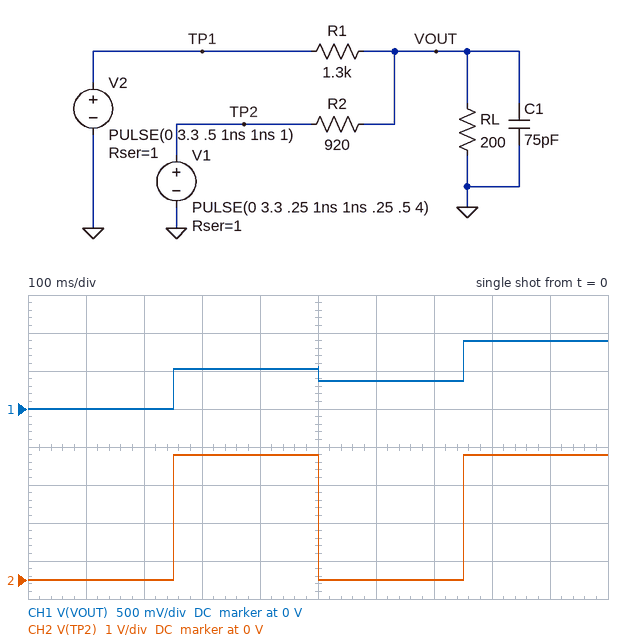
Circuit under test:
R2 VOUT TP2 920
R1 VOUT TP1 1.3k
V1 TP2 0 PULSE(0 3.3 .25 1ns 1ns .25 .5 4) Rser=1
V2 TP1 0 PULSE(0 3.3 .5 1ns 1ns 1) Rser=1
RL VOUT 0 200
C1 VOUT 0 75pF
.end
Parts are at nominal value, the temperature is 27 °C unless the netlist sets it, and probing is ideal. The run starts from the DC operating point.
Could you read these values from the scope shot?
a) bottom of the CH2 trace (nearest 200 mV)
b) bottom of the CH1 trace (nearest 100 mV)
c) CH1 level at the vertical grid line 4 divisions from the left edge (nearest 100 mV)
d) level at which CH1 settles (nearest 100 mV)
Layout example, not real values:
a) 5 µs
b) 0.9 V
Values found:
a) 0 V
b) 0 V
c) 500 mV
d) 900 mV
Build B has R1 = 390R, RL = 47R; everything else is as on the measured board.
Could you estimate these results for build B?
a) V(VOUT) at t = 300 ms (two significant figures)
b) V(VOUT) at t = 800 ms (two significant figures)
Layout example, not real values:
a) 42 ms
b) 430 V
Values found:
a) 140 mV
b) 480 mV
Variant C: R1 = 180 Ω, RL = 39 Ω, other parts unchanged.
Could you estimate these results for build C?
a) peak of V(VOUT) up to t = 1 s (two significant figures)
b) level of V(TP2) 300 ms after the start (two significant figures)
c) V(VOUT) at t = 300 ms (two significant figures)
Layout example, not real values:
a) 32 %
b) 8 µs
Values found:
a) 680 mV
b) 3.3 V
c) 110 mV
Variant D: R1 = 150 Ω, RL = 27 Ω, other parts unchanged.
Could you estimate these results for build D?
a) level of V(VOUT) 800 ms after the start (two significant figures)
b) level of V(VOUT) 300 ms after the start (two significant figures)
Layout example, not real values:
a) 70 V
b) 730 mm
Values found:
a) 570 mV
b) 80 mV
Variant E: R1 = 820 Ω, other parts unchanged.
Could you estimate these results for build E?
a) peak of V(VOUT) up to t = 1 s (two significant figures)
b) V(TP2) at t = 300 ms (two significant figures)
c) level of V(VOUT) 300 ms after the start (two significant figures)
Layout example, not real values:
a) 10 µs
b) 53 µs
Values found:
a) 1.0 V
b) 3.3 V
c) 490 mV
